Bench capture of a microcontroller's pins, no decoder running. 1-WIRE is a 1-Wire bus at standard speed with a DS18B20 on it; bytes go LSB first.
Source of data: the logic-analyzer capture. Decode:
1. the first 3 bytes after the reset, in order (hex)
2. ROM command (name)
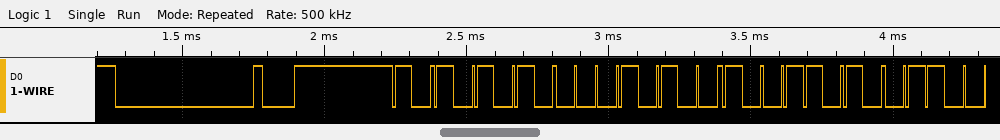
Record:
55 28 59
Match ROM
